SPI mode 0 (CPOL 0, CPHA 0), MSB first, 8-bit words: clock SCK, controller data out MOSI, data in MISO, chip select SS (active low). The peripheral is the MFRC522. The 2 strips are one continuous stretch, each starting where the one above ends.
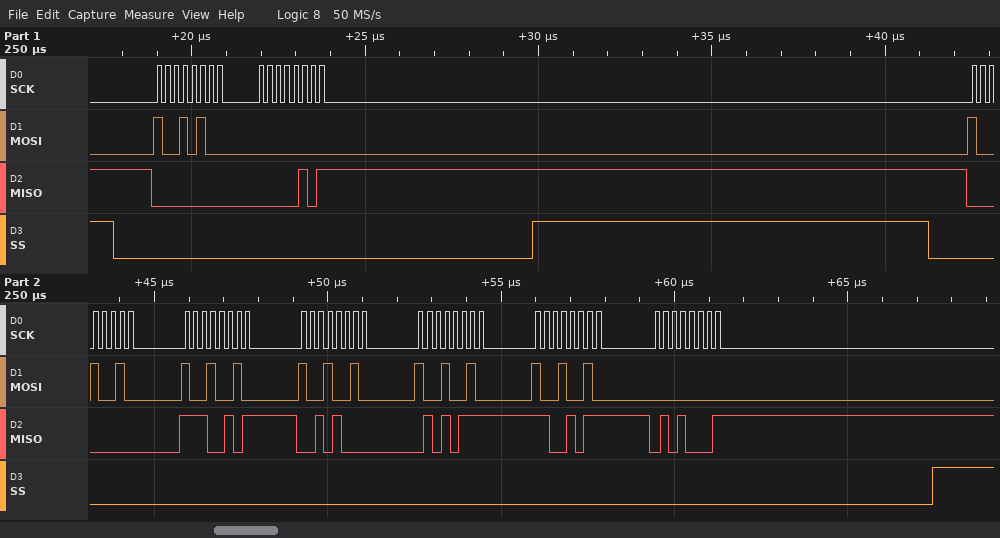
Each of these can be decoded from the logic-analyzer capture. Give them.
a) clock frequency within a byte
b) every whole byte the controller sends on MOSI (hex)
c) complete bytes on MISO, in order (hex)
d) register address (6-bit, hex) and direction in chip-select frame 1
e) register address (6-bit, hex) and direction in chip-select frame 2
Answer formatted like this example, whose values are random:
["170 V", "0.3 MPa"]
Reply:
["4 MHz", "94 00 92 92 92 92 92 00", "00 05 00 E5 28 57 CB 51", "0x0A read", "0x09 read"]
